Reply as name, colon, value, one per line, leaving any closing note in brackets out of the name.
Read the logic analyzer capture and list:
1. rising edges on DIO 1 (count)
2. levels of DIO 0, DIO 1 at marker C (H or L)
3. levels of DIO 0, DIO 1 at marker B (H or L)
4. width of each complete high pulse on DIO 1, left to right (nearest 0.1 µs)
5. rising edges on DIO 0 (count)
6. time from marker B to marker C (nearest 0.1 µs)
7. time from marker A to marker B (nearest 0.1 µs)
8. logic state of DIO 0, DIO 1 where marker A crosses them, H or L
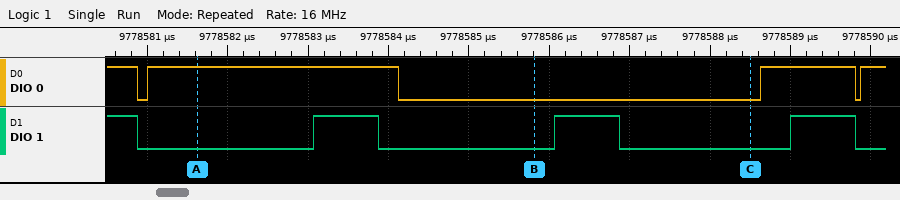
rising edges on DIO 1: 3
levels of DIO 0, DIO 1 at marker C: DIO 0=L, DIO 1=L
levels of DIO 0, DIO 1 at marker B: DIO 0=L, DIO 1=L
width of each complete high pulse on DIO 1, left to right: 0.8 µs, 0.8 µs, 0.8 µs
rising edges on DIO 0: 3
time from marker B to marker C: 2.7 µs
time from marker A to marker B: 4.2 µs
logic state of DIO 0, DIO 1 where marker A crosses them, H or L: DIO 0=H, DIO 1=L
